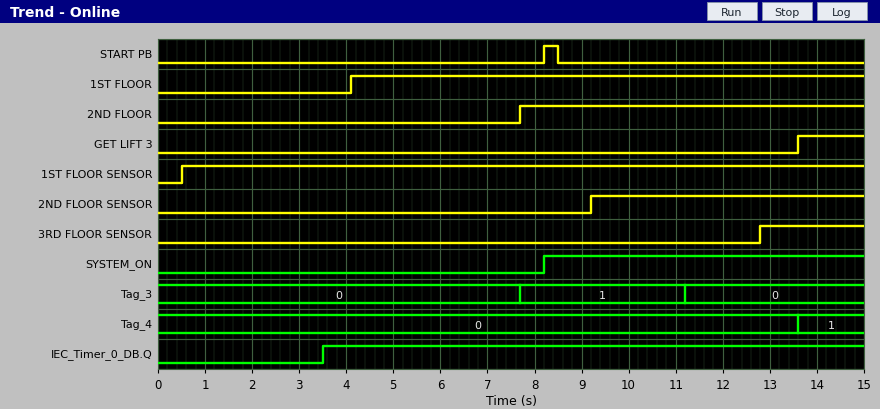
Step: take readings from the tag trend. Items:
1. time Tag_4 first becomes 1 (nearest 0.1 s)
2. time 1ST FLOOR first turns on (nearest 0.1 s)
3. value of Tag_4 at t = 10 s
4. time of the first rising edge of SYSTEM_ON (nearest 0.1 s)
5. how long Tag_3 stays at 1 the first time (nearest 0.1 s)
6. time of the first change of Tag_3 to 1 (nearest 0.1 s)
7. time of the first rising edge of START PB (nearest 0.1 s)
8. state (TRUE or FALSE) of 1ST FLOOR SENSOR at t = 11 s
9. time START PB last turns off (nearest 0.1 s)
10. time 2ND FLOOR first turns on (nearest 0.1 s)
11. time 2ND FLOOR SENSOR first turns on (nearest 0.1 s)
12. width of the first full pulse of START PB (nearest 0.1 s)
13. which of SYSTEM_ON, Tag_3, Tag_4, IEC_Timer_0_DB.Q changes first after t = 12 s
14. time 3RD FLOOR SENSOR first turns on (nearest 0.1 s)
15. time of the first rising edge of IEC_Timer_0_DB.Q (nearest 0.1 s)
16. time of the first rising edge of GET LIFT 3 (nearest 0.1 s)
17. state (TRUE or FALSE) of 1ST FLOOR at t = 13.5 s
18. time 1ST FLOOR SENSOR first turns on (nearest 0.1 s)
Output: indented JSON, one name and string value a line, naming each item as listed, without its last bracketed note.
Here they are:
{
  "time Tag_4 first becomes 1": "13.6 s",
  "time 1ST FLOOR first turns on": "4.1 s",
  "value of Tag_4 at t = 10 s": "0",
  "time of the first rising edge of SYSTEM_ON": "8.2 s",
  "how long Tag_3 stays at 1 the first time": "3.5 s",
  "time of the first change of Tag_3 to 1": "7.7 s",
  "time of the first rising edge of START PB": "8.2 s",
  "state (TRUE or FALSE) of 1ST FLOOR SENSOR at t = 11 s": "TRUE",
  "time START PB last turns off": "8.5 s",
  "time 2ND FLOOR first turns on": "7.7 s",
  "time 2ND FLOOR SENSOR first turns on": "9.2 s",
  "width of the first full pulse of START PB": "0.3 s",
  "which of SYSTEM_ON, Tag_3, Tag_4, IEC_Timer_0_DB.Q changes first after t = 12 s": "Tag_4",
  "time 3RD FLOOR SENSOR first turns on": "12.8 s",
  "time of the first rising edge of IEC_Timer_0_DB.Q": "3.5 s",
  "time of the first rising edge of GET LIFT 3": "13.6 s",
  "state (TRUE or FALSE) of 1ST FLOOR at t = 13.5 s": "TRUE",
  "time 1ST FLOOR SENSOR first turns on": "0.5 s"
}
